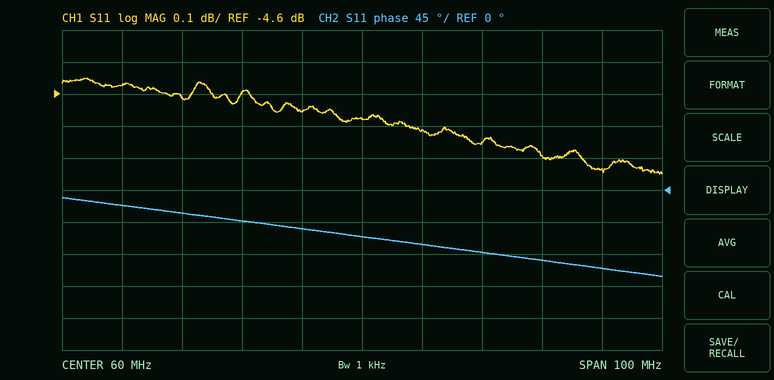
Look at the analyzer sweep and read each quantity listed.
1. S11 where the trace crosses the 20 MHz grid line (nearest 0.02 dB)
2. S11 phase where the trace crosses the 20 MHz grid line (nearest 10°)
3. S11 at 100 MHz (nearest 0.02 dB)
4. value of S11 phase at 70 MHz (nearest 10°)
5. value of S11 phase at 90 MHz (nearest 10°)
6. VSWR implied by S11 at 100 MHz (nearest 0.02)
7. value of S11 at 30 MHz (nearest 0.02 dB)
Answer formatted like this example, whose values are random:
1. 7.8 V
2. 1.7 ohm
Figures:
1. -4.58 dB
2. -20°
3. -4.84 dB
4. -80°
5. -100°
6. 3.68
7. -4.62 dB
